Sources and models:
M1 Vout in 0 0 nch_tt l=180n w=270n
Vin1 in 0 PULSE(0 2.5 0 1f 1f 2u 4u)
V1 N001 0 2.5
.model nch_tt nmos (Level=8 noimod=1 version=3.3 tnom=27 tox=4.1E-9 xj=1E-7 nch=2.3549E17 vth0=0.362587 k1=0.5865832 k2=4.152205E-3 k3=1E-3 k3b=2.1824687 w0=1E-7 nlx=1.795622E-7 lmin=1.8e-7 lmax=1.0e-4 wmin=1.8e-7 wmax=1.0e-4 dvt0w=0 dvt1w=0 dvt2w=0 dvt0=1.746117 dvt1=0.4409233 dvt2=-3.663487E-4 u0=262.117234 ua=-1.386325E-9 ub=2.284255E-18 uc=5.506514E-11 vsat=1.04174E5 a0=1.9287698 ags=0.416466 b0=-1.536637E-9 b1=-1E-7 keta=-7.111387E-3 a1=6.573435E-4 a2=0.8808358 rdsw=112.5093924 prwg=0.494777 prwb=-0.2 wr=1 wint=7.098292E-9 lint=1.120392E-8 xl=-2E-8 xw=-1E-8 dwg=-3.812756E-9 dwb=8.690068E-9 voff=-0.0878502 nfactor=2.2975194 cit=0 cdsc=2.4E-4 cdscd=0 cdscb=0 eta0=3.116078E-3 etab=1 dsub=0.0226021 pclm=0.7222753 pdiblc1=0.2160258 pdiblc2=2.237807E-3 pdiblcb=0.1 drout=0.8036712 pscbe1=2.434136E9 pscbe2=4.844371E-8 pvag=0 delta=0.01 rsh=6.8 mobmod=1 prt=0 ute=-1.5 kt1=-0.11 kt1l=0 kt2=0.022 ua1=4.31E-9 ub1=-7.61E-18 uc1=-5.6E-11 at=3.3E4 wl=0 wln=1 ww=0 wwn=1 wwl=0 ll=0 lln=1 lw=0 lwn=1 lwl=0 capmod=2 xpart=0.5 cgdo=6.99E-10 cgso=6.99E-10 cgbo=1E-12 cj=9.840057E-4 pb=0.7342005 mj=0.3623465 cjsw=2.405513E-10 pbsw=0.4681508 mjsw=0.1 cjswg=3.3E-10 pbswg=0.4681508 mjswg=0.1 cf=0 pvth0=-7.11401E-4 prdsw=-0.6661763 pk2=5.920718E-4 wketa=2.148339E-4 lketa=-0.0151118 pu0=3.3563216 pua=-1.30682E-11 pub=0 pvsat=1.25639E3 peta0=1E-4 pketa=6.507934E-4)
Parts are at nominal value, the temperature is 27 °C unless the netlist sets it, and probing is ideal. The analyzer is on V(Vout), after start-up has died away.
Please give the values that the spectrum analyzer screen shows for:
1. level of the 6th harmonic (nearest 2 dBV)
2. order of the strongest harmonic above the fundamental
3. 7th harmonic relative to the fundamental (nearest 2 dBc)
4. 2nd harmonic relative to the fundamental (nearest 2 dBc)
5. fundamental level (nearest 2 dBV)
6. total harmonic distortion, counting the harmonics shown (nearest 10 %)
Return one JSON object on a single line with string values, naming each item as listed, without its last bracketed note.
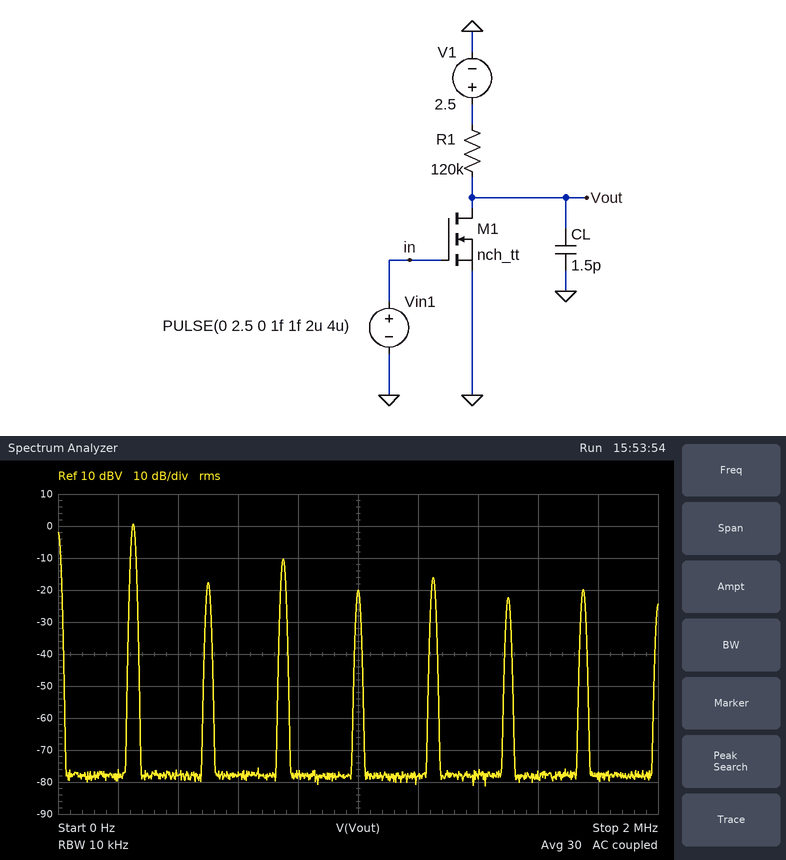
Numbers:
{"level of the 6th harmonic": "-22 dBV", "order of the strongest harmonic above the fundamental": "3", "7th harmonic relative to the fundamental": "-20 dBc", "2nd harmonic relative to the fundamental": "-18 dBc", "fundamental level": "0 dBV", "total harmonic distortion, counting the harmonics shown": "40 %"}
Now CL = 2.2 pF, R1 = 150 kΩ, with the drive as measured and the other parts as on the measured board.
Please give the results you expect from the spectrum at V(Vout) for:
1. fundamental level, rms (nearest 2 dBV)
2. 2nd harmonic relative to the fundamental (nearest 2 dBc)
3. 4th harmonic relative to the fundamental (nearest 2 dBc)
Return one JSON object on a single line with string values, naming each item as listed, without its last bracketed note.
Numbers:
{"fundamental level, rms": "0 dBV", "2nd harmonic relative to the fundamental": "-14 dBc", "4th harmonic relative to the fundamental": "-18 dBc"}
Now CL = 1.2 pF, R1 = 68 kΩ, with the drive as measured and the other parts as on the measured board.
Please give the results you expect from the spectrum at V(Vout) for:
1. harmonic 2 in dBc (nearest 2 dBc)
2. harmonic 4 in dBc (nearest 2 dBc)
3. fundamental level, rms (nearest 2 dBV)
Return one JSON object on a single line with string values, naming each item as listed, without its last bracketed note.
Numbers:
{"harmonic 2 in dBc": "-24 dBc", "harmonic 4 in dBc": "-26 dBc", "fundamental level, rms": "0 dBV"}
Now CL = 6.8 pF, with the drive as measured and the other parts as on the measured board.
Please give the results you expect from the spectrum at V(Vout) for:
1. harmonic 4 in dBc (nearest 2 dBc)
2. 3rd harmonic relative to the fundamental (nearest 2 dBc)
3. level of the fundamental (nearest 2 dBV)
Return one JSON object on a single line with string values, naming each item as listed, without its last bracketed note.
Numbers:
{"harmonic 4 in dBc": "-16 dBc", "3rd harmonic relative to the fundamental": "-12 dBc", "level of the fundamental": "-2 dBV"}
